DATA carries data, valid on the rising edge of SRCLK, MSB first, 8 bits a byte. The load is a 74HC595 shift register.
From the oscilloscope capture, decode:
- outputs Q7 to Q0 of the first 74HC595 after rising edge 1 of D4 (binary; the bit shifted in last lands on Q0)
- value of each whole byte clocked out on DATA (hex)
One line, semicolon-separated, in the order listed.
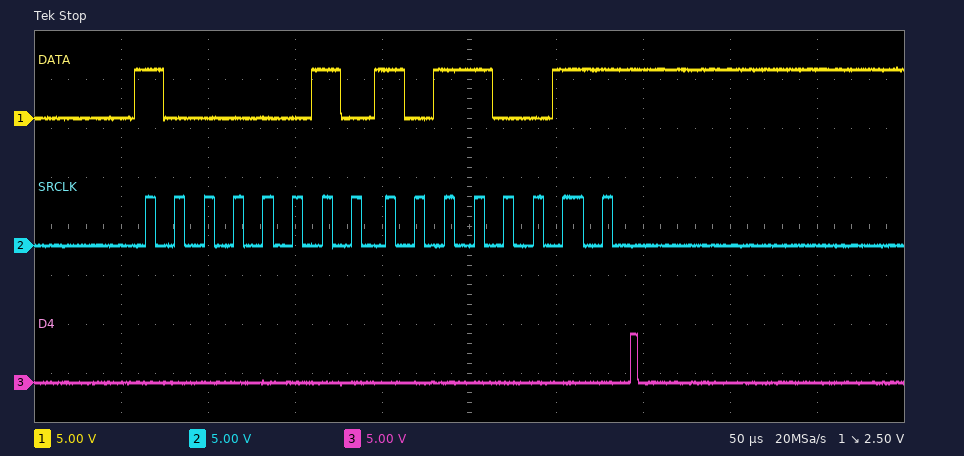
10110011; 82 B3
